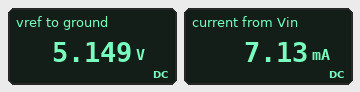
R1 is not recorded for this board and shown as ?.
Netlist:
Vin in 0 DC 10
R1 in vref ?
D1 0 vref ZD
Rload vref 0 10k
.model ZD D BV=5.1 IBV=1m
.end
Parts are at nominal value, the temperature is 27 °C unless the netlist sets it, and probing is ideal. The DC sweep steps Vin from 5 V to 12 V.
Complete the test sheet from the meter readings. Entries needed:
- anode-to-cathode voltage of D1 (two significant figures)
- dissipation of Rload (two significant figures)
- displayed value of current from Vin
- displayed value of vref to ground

-5.1 V
2.7 mW
7.13 mA
5.149 V
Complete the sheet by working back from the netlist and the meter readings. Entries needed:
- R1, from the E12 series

680 Ω
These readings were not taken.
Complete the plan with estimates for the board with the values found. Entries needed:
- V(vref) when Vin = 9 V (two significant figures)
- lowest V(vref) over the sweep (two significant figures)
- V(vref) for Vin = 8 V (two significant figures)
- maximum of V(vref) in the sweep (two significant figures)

5.1 V
4.7 V
5.1 V
5.2 V
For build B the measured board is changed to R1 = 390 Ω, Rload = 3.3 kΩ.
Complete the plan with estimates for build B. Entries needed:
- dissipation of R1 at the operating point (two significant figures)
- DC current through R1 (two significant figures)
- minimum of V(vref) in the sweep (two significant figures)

60 mW
12 mA
4.5 V
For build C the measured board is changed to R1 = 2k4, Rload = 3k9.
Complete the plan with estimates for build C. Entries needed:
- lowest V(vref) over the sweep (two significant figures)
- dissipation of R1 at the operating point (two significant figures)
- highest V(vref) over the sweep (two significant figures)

3.1 V
10 mW
5.1 V
